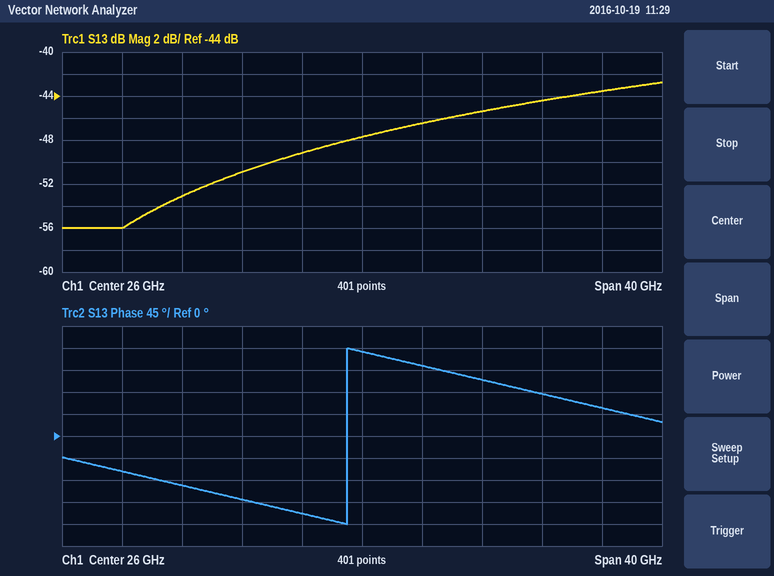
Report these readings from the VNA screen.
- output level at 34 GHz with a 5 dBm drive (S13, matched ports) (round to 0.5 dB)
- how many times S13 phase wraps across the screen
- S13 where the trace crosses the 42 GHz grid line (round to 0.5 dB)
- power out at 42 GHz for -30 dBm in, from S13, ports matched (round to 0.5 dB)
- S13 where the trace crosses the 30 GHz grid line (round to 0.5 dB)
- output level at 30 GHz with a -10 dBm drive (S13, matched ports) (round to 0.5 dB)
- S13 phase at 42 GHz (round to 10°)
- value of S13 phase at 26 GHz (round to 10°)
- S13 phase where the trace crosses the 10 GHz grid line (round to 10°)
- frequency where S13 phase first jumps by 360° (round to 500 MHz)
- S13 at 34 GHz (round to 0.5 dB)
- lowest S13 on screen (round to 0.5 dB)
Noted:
-40.5 dBm
1
-43.5 dB
-73.5 dBm
-46.5 dB
-56.5 dBm
60°
170°
-70°
25.0 GHz
-45.5 dB
-56.0 dB
